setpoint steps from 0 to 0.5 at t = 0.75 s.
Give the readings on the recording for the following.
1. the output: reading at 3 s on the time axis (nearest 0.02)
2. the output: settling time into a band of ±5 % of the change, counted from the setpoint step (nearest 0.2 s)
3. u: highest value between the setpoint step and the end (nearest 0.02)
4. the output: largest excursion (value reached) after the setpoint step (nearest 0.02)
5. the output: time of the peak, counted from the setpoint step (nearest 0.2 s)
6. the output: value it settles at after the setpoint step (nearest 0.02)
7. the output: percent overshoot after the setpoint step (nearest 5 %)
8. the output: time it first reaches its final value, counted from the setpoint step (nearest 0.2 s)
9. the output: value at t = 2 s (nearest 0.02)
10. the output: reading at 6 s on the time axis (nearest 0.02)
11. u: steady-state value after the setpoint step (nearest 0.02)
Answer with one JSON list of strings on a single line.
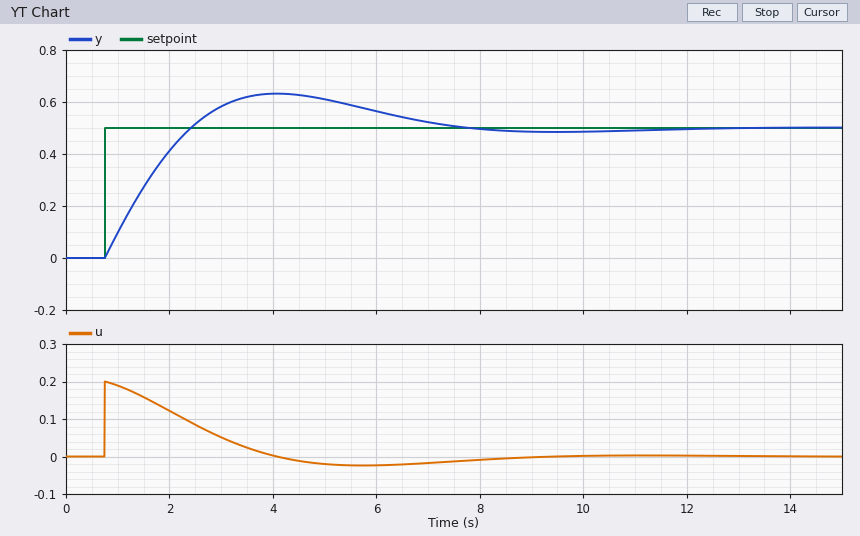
["0.58", "6.2 s", "0.20", "0.64", "3.4 s", "0.50", "25 %", "1.6 s", "0.42", "0.56", "0.00"]
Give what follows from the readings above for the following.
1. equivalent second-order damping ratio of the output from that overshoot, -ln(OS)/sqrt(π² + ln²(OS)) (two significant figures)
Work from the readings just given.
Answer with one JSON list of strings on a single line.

["0.40"]
